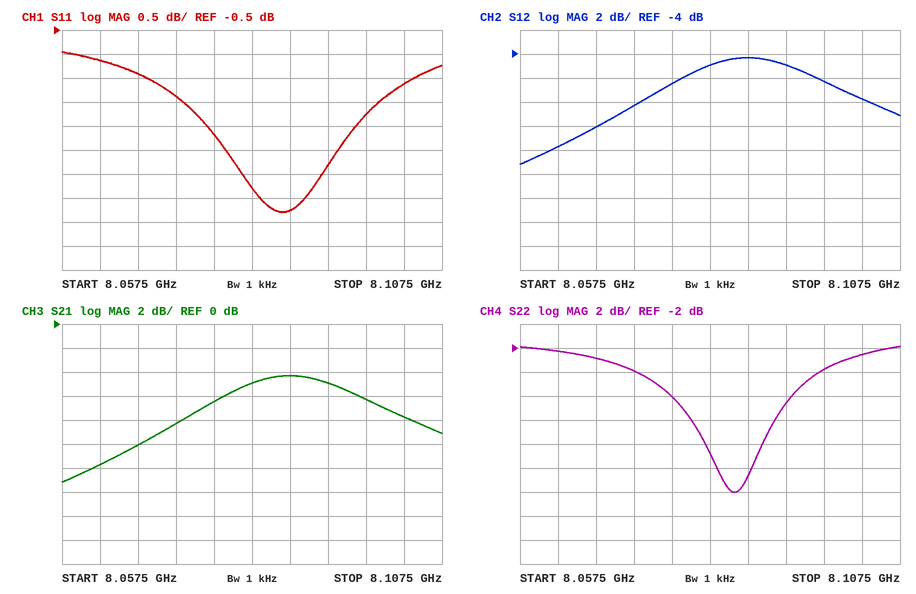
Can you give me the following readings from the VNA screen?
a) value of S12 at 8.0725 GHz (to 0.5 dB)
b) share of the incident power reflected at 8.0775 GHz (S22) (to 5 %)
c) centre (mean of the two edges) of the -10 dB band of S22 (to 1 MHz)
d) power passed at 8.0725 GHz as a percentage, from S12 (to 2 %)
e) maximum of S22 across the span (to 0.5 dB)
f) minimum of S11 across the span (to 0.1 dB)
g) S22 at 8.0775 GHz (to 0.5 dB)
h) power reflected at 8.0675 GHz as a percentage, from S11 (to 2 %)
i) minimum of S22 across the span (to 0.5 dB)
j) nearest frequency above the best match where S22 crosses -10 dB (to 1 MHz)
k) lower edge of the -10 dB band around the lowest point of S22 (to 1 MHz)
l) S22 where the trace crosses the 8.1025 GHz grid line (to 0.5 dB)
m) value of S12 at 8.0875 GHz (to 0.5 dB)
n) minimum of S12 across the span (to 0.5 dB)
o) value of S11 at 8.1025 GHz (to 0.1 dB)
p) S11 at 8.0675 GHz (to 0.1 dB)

-8.5 dB
25 %
8.086 GHz
14 %
-2.0 dB
-4.3 dB
-6.0 dB
72 %
-14.0 dB
8.089 GHz
8.082 GHz
-2.5 dB
-4.5 dB
-13.0 dB
-1.6 dB
-1.4 dB
